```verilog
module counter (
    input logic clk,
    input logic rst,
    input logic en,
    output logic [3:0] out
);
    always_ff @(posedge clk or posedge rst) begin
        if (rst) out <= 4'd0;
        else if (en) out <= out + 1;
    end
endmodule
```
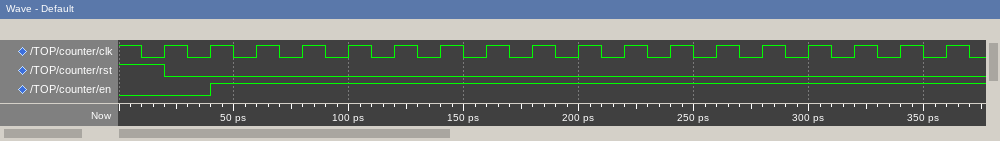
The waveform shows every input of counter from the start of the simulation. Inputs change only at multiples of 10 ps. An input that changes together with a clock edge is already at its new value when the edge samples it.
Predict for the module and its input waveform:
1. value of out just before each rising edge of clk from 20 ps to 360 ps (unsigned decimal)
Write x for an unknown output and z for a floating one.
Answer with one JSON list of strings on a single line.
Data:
["0, 0, 1, 2, 3, 4, 5, 6, 7, 8, 9, 10, 11, 12, 13, 14, 15, 0"]
